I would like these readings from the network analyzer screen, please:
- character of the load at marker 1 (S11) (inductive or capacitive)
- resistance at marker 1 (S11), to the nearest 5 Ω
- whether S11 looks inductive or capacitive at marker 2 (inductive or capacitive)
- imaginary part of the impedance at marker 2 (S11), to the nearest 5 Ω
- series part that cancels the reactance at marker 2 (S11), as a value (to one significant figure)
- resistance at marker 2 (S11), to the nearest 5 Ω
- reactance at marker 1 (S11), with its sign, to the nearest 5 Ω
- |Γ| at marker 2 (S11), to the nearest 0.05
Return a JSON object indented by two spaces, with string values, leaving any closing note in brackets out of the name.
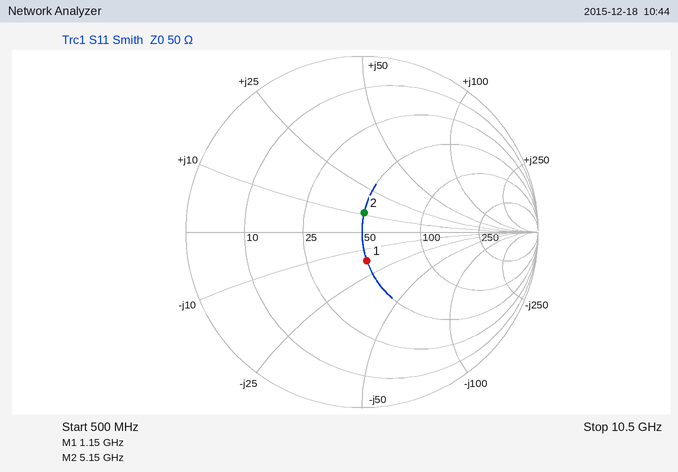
{
  "character of the load at marker 1 (S11)": "capacitive",
  "resistance at marker 1 (S11), to the nearest 5 Ω": "50 Ω",
  "whether S11 looks inductive or capacitive at marker 2": "inductive",
  "imaginary part of the impedance at marker 2 (S11), to the nearest 5 Ω": "+10 Ω",
  "series part that cancels the reactance at marker 2 (S11), as a value": "3 pF",
  "resistance at marker 2 (S11), to the nearest 5 Ω": "50 Ω",
  "reactance at marker 1 (S11), with its sign, to the nearest 5 Ω": "-15 Ω",
  "|Γ| at marker 2 (S11), to the nearest 0.05": "0.10"
}
